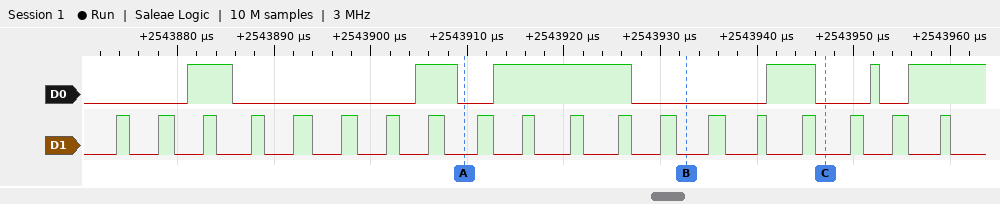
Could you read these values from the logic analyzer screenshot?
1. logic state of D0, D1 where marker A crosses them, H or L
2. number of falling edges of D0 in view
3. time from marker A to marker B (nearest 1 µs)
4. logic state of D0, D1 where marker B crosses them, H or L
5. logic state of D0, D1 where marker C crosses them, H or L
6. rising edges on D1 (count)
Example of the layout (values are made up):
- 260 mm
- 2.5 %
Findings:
- D0=L, D1=L
- 5
- 23 µs
- D0=L, D1=L
- D0=L, D1=L
- 19
